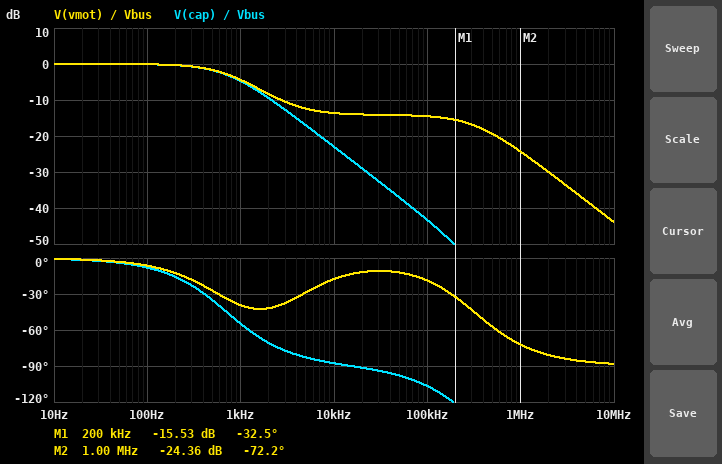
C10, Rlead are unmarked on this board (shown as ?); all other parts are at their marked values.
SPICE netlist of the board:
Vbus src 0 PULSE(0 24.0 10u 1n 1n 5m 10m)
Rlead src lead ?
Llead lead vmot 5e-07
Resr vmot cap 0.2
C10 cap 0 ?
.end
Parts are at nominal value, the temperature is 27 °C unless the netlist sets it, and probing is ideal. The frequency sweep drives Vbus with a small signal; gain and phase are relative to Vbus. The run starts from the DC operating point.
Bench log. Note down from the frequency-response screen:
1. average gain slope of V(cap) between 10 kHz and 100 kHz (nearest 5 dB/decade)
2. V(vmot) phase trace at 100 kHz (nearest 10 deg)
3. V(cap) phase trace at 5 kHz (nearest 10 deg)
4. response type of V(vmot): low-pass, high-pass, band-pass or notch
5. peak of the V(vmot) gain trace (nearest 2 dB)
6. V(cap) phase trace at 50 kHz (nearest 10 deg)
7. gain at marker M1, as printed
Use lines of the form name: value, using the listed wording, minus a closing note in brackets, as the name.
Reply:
average gain slope of V(cap) between 10 kHz and 100 kHz: -20 dB/decade
V(vmot) phase trace at 100 kHz: -20 deg
V(cap) phase trace at 5 kHz: -80 deg
response type of V(vmot): low-pass, high-pass, band-pass or notch: low-pass
peak of the V(vmot) gain trace: 0 dB
V(cap) phase trace at 50 kHz: -100 deg
gain at marker M1, as printed: -15.53 dB
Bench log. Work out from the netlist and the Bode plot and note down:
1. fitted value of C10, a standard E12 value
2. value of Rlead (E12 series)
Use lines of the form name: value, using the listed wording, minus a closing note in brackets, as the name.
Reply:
fitted value of C10, a standard E12 value: 220 µF
value of Rlead: 0.82 Ω
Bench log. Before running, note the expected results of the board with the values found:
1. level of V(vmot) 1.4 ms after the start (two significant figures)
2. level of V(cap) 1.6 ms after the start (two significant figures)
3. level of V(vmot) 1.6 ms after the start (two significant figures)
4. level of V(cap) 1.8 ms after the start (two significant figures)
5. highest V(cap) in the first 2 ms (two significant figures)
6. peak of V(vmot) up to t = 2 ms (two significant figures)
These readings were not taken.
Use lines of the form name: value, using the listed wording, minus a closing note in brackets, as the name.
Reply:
level of V(vmot) 1.4 ms after the start: 24 V
level of V(cap) 1.6 ms after the start: 24 V
level of V(vmot) 1.6 ms after the start: 24 V
level of V(cap) 1.8 ms after the start: 24 V
highest V(cap) in the first 2 ms: 24 V
peak of V(vmot) up to t = 2 ms: 24 V
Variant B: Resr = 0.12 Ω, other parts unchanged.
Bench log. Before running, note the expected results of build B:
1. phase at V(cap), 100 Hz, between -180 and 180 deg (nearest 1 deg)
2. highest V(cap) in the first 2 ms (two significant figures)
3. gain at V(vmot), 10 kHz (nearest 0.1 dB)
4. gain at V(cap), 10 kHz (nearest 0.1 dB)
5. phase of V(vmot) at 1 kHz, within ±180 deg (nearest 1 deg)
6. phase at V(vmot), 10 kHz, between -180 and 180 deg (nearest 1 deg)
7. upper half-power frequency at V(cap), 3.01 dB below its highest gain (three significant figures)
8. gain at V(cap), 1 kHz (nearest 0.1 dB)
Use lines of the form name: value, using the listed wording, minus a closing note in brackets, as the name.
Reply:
phase at V(cap), 100 Hz, between -180 and 180 deg: -7 deg
highest V(cap) in the first 2 ms: 24 V
gain at V(vmot), 10 kHz: -16.5 dB
gain at V(cap), 10 kHz: -22.3 dB
phase of V(vmot) at 1 kHz, within ±180 deg: -43 deg
phase at V(vmot), 10 kHz, between -180 and 180 deg: -29 deg
upper half-power frequency at V(cap), 3.01 dB below its highest gain: 772 Hz
gain at V(cap), 1 kHz: -4.3 dB
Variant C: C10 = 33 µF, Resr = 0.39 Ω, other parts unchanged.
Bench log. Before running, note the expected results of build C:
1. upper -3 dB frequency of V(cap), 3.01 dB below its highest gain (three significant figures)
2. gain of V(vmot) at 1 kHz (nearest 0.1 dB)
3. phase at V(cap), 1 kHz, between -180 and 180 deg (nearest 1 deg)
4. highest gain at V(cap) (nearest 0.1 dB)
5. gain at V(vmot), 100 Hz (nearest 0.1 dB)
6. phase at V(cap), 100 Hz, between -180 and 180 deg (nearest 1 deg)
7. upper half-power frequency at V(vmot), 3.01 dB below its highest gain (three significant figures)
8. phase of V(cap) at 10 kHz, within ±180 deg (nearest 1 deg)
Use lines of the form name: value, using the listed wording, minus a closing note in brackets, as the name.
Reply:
upper -3 dB frequency of V(cap), 3.01 dB below its highest gain: 4.03 kHz
gain of V(vmot) at 1 kHz: -0.2 dB
phase at V(cap), 1 kHz, between -180 and 180 deg: -14 deg
highest gain at V(cap): 0 dB
gain at V(vmot), 100 Hz: 0 dB
phase at V(cap), 100 Hz, between -180 and 180 deg: -1 deg
upper half-power frequency at V(vmot), 3.01 dB below its highest gain: 4.54 kHz
phase of V(cap) at 10 kHz, within ±180 deg: -70 deg
